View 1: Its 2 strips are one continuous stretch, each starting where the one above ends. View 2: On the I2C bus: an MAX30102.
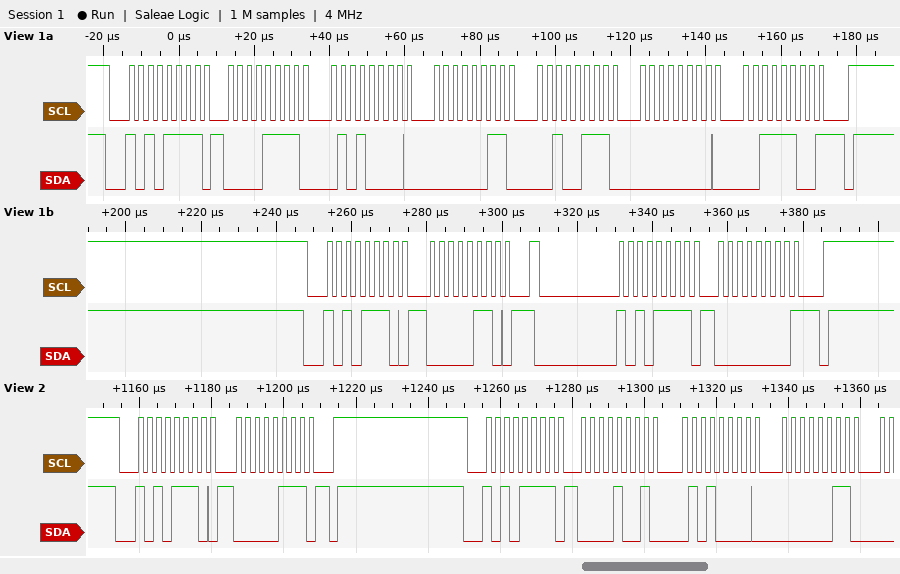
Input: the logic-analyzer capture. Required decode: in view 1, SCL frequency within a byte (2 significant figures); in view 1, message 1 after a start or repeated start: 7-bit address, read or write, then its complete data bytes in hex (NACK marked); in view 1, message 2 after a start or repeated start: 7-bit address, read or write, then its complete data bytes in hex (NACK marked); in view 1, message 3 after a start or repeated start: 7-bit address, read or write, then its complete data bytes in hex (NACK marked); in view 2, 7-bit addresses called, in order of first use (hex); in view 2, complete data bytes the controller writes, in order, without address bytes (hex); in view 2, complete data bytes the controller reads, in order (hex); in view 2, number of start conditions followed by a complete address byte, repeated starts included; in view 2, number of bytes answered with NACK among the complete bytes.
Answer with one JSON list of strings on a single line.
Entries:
["400 kHz", "0x57 read: 0F 50 03 27 00 3C NACK", "0x57 write: 06", "0x57 read: 00 NACK", "0x57", "07", "09 50 03", "2", "0"]
